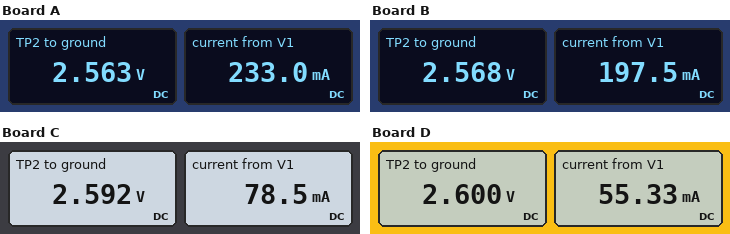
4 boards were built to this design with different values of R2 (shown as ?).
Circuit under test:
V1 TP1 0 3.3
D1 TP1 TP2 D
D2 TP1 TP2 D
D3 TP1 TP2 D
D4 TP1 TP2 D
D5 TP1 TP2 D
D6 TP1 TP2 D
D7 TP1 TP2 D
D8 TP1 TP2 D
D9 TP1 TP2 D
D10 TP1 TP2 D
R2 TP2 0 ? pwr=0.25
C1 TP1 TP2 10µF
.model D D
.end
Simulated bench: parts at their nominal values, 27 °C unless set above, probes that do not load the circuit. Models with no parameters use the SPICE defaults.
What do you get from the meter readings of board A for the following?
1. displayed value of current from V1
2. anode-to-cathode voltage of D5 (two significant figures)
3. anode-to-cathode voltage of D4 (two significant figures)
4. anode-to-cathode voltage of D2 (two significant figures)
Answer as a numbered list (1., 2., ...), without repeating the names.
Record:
1. 233.0 mA
2. 740 mV
3. 740 mV
4. 740 mV
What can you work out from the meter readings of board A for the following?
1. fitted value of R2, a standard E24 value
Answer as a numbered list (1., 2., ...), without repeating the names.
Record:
1. 11 Ω
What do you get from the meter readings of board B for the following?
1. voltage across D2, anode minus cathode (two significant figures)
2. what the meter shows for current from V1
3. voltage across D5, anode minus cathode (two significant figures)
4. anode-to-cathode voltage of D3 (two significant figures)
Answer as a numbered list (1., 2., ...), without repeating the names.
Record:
1. 730 mV
2. 197.5 mA
3. 730 mV
4. 730 mV
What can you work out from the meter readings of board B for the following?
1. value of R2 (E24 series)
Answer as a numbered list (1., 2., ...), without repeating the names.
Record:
1. 13 Ω
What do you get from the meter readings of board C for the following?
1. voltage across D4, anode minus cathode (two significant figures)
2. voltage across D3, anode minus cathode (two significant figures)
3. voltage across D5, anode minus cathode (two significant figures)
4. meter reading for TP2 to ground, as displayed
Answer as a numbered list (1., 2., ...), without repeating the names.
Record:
1. 710 mV
2. 710 mV
3. 710 mV
4. 2.592 V
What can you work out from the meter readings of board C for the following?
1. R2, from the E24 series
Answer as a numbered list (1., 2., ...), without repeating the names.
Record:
1. 33 Ω
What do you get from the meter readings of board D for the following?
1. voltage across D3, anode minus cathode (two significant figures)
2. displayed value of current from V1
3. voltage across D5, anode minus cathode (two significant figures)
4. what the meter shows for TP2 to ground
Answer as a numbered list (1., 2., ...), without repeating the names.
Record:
1. 700 mV
2. 55.33 mA
3. 700 mV
4. 2.600 V
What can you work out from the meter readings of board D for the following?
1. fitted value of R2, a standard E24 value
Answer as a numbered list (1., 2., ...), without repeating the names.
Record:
1. 47 Ω
